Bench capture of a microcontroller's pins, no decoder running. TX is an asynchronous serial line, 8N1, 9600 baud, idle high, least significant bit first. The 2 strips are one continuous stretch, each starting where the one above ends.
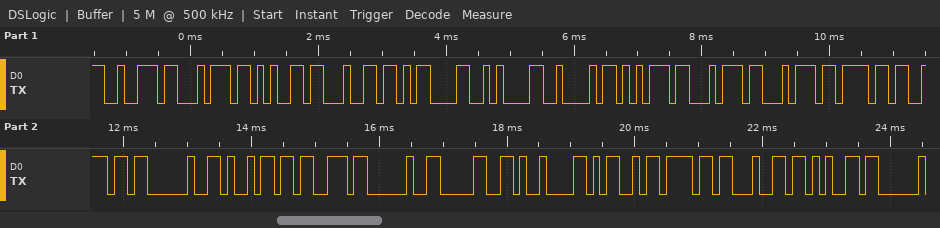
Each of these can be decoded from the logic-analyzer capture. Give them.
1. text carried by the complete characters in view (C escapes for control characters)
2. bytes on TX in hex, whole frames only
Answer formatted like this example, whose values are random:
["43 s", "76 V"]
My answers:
["\"rted\\r\\nButton is 0\\tMode\"", "72 74 65 64 0D 0A 42 75 74 74 6F 6E 20 69 73 20 30 09 4D 6F 64 65"]
